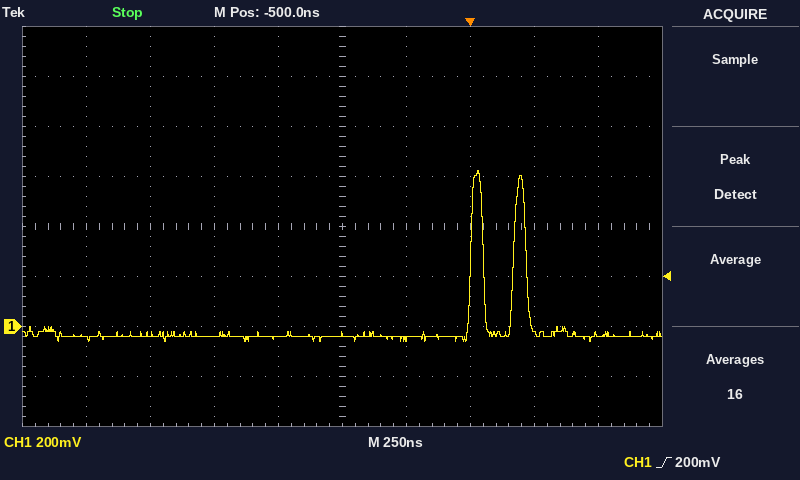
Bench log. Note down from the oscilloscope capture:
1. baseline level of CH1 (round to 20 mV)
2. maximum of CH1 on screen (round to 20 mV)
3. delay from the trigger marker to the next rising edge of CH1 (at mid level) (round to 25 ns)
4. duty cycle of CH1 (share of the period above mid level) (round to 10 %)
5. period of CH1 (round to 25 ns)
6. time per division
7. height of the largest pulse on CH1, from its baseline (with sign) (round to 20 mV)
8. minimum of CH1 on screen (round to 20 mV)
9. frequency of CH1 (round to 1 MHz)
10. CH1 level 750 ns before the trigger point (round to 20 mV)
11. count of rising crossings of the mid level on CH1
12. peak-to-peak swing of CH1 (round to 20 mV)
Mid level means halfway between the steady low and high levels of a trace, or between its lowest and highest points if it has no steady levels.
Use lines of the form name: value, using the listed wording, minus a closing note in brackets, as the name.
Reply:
baseline level of CH1: -40 mV
maximum of CH1 on screen: 620 mV
delay from the trigger marker to the next rising edge of CH1 (at mid level): 175 ns
duty cycle of CH1 (share of the period above mid level): 30 %
period of CH1: 175 ns
time per division: 250 ns
height of the largest pulse on CH1, from its baseline (with sign): +660 mV
minimum of CH1 on screen: -60 mV
frequency of CH1: 6 MHz
CH1 level 750 ns before the trigger point: -40 mV
count of rising crossings of the mid level on CH1: 2
peak-to-peak swing of CH1: 680 mV
